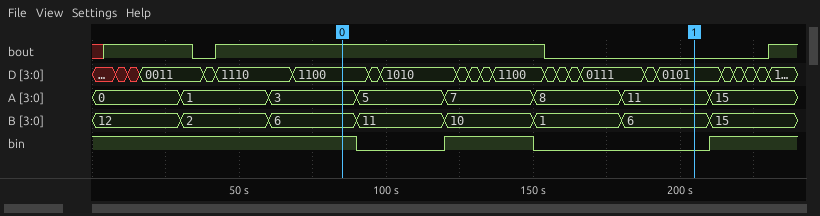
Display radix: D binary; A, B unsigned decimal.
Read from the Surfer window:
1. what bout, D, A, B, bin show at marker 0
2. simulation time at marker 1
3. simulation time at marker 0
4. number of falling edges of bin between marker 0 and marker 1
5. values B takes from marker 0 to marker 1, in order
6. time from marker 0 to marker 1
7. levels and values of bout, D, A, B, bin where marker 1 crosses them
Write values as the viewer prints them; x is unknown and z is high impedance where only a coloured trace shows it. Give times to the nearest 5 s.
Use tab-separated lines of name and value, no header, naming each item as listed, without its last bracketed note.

what bout, D, A, B, bin show at marker 0	bout=1, D=1100, A=3, B=6, bin=1
simulation time at marker 1	205 s
simulation time at marker 0	85 s
number of falling edges of bin between marker 0 and marker 1	2
values B takes from marker 0 to marker 1, in order	6, 11, 10, 1, 6
time from marker 0 to marker 1	120 s
levels and values of bout, D, A, B, bin where marker 1 crosses them	bout=0, D=0101, A=11, B=6, bin=0
